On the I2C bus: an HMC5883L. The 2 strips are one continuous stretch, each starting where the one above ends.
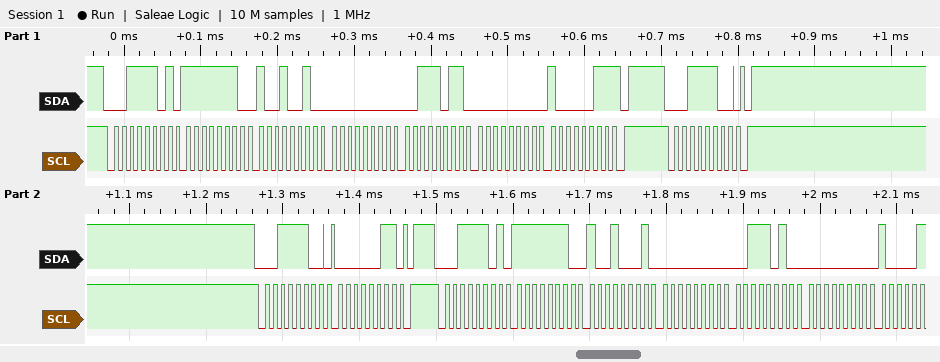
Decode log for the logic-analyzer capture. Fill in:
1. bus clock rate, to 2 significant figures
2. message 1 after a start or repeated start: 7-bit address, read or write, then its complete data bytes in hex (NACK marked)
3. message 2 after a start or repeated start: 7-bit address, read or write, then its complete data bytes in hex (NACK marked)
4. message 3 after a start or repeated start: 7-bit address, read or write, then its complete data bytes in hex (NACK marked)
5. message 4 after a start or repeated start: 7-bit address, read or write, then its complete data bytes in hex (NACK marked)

100 kHz
0x1E read: FE 92 00 3B 00 83 NACK
0x1E write
0x1E write: 03
0x1E read: FE 91 00 3A 00
